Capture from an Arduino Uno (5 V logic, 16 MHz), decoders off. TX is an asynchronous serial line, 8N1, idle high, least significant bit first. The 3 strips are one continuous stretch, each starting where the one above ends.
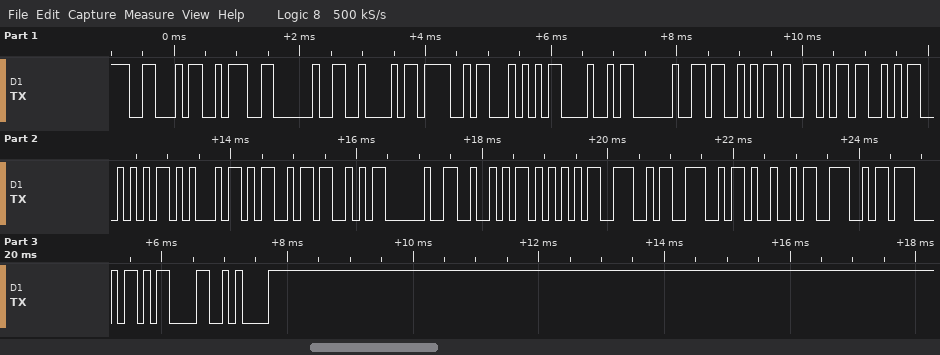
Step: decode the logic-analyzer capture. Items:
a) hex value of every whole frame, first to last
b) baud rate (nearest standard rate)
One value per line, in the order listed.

46 3A 20 42 4F 54 48 20 53 59 53 54 45 4D 53 20 52 55 4E 4E 49 4E 47 0D 0A
9600 baud
